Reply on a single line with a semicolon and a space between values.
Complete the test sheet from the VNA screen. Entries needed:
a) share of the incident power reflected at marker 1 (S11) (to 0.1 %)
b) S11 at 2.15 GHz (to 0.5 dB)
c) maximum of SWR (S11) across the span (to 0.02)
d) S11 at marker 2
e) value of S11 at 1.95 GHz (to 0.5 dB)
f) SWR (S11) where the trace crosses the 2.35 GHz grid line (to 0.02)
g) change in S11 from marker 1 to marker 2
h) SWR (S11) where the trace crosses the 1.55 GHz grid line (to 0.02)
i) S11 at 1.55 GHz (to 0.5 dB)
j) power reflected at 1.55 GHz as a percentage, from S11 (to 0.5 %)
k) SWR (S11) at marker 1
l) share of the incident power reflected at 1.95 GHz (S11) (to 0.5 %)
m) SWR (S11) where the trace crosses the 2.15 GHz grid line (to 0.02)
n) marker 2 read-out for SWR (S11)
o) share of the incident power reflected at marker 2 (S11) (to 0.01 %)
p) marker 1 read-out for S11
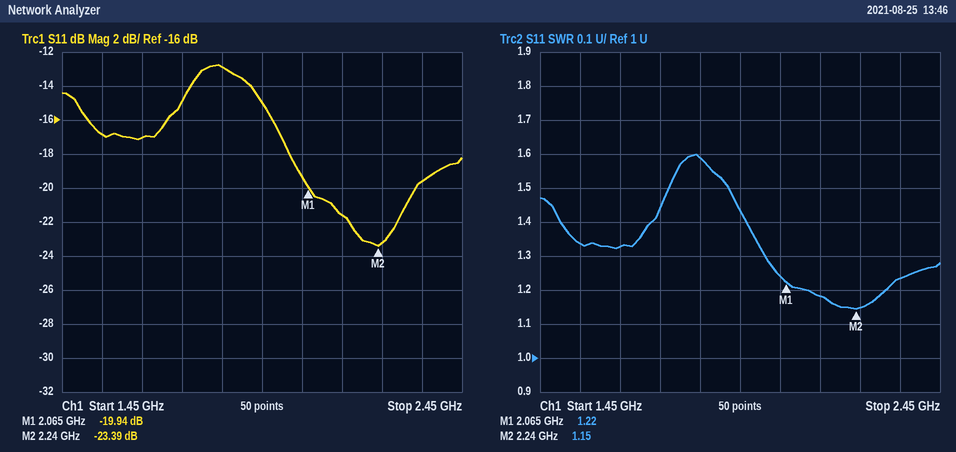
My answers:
1.0 %; -21.5 dB; 1.60; -23.39 dB; -15.0 dB; 1.24; -3.45 dB; 1.34; -17.0 dB; 2.0 %; 1.22; 3.0 %; 1.18; 1.15; 0.46 %; -19.94 dB
